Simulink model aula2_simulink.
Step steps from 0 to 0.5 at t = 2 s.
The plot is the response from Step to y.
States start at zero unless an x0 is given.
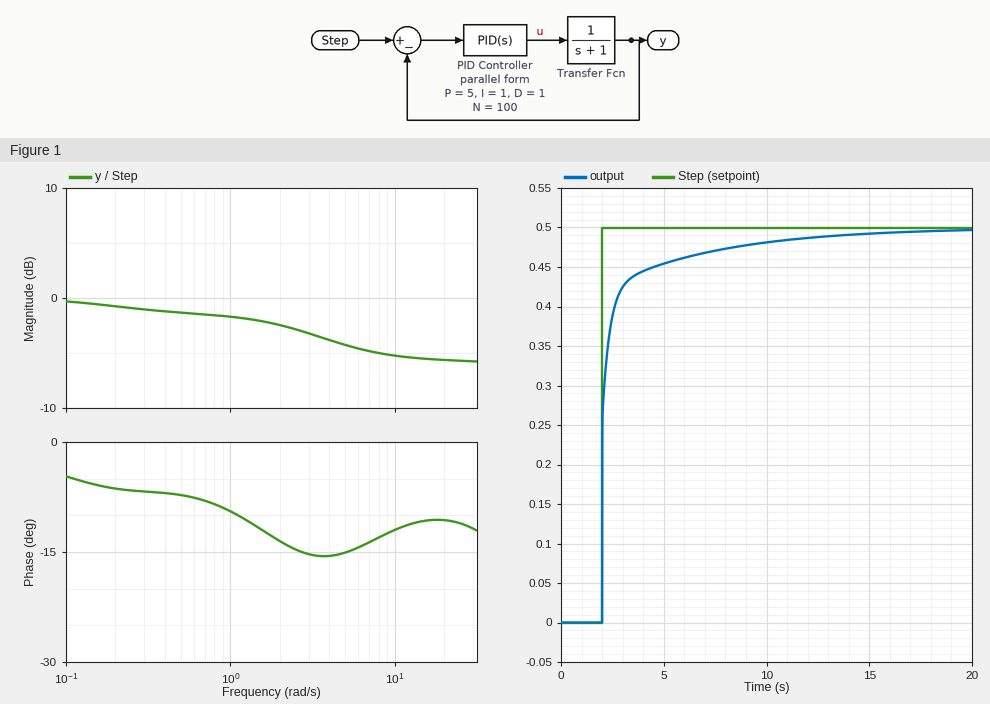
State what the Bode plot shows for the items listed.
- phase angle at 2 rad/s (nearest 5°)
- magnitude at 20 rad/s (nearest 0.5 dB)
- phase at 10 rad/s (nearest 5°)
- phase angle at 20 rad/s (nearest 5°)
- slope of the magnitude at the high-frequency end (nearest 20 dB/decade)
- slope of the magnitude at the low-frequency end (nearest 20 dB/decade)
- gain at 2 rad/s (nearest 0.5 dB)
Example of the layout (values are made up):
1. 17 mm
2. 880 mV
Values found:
1. -15°
2. -5.5 dB
3. -10°
4. -10°
5. 0 dB/decade
6. 0 dB/decade
7. -2.5 dB
